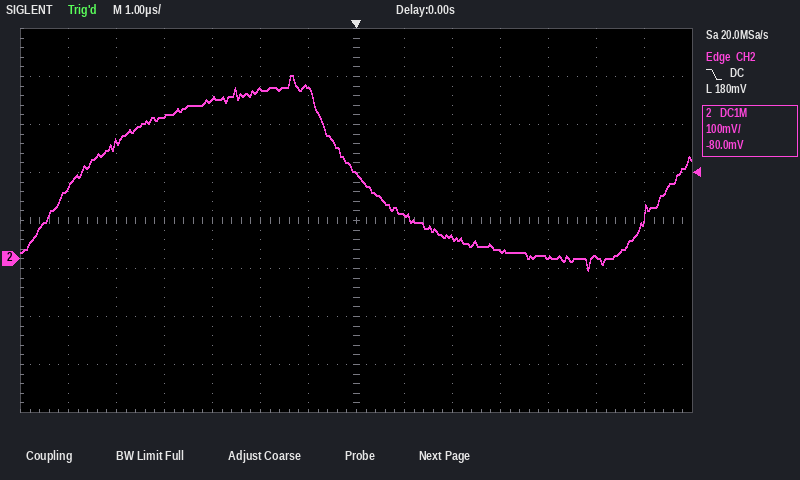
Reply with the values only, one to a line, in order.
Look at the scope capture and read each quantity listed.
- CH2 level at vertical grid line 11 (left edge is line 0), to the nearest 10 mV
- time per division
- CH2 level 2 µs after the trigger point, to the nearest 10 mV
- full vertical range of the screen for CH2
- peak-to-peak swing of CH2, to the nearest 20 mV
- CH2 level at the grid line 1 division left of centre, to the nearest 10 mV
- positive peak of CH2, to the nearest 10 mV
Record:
0 mV
1 µs
40 mV
800 mV
400 mV
360 mV
380 mV
